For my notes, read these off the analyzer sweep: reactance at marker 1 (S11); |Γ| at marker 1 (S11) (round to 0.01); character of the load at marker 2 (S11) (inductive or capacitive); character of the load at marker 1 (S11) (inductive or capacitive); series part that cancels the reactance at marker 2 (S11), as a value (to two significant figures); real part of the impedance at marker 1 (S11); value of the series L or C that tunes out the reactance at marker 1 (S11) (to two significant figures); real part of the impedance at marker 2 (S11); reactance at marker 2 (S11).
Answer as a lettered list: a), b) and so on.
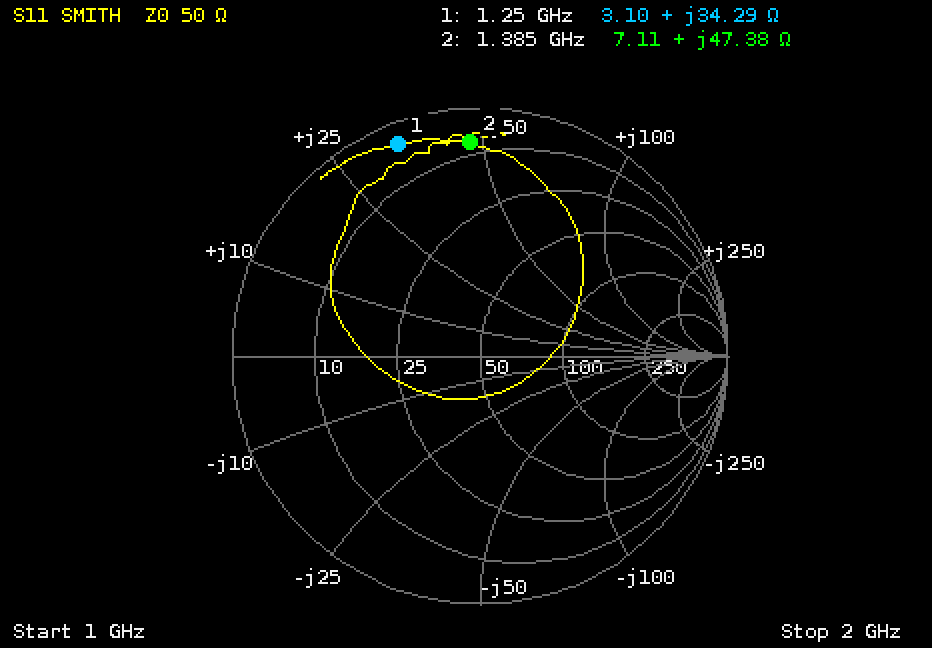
a) +34.29 Ω
b) 0.92
c) inductive
d) inductive
e) 2.4 pF
f) 3.10 Ω
g) 3.7 pF
h) 7.11 Ω
i) +47.38 Ω
